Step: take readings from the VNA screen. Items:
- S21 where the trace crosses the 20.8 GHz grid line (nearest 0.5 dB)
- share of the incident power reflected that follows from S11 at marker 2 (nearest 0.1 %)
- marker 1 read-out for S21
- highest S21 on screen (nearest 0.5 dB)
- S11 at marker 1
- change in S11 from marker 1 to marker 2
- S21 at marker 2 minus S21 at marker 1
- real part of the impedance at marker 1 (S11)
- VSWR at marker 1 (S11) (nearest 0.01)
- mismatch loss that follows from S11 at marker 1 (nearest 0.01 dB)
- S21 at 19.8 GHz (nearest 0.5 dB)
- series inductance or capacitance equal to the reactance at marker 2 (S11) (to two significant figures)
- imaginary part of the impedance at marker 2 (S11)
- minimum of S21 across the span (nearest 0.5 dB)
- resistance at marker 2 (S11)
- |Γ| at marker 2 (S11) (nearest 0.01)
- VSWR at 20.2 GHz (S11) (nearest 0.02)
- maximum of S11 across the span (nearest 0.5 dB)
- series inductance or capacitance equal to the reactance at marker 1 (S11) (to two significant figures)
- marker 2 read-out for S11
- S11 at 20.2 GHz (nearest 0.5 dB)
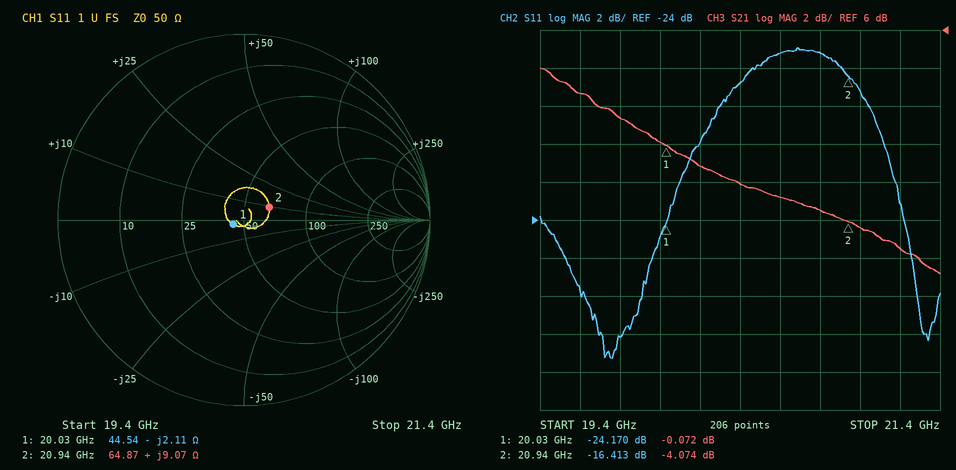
-3.5 dB
2.3 %
-0.072 dB
4.0 dB
-24.170 dB
7.757 dB
-4.002 dB
44.54 Ω
1.13
0.02 dB
1.5 dB
69 pH
+9.07 Ω
-7.0 dB
64.87 Ω
0.15
1.22
-15.0 dB
3.8 pF
-16.413 dB
-20.0 dB
